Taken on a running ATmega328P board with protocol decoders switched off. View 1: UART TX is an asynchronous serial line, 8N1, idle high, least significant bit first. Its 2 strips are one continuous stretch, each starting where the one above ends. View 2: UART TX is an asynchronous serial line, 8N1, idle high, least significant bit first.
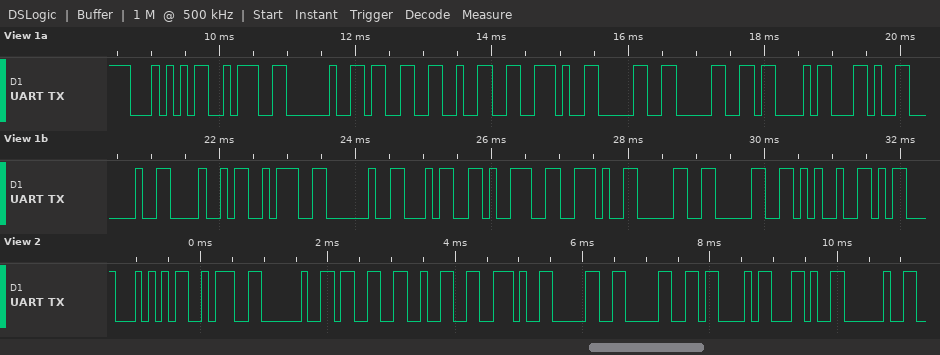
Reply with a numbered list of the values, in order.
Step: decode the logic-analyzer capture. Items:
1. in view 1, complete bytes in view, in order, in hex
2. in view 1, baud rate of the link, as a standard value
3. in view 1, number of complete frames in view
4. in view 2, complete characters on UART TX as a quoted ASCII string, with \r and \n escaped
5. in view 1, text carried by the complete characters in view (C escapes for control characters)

1. 54 3A 20 33 32 2E 30 30 43 2C 20 48 3A 20 34 39 2E 30 30 25
2. 9600 baud
3. 20
4. "T: 32.00C, "
5. "T: 32.00C, H: 49.00%"
